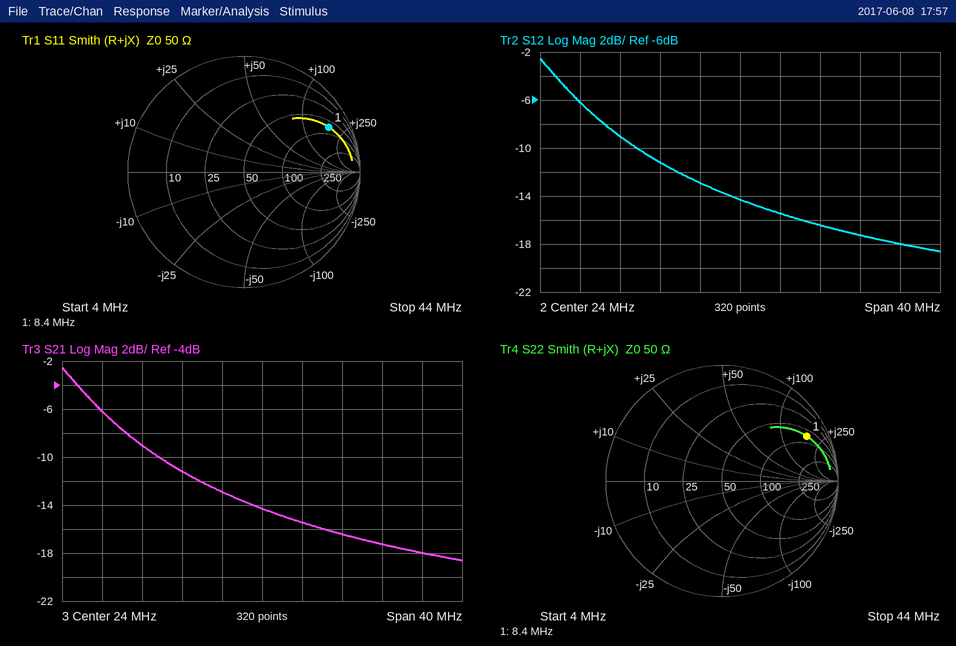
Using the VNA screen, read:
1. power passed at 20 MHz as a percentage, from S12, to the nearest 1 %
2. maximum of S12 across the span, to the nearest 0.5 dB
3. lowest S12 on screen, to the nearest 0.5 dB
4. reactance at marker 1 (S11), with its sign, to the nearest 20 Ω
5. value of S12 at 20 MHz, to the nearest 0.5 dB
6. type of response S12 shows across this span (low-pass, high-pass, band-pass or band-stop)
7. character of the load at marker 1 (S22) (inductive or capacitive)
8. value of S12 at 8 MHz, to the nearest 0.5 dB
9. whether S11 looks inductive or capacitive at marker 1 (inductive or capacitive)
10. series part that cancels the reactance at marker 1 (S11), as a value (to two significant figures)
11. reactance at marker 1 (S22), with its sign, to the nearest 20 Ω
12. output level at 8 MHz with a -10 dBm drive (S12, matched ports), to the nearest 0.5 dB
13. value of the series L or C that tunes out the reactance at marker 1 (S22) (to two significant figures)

5 %
-2.5 dB
-18.5 dB
+180 Ω
-13.0 dB
low-pass
inductive
-6.0 dB
inductive
110 pF
+180 Ω
-16.0 dBm
110 pF
